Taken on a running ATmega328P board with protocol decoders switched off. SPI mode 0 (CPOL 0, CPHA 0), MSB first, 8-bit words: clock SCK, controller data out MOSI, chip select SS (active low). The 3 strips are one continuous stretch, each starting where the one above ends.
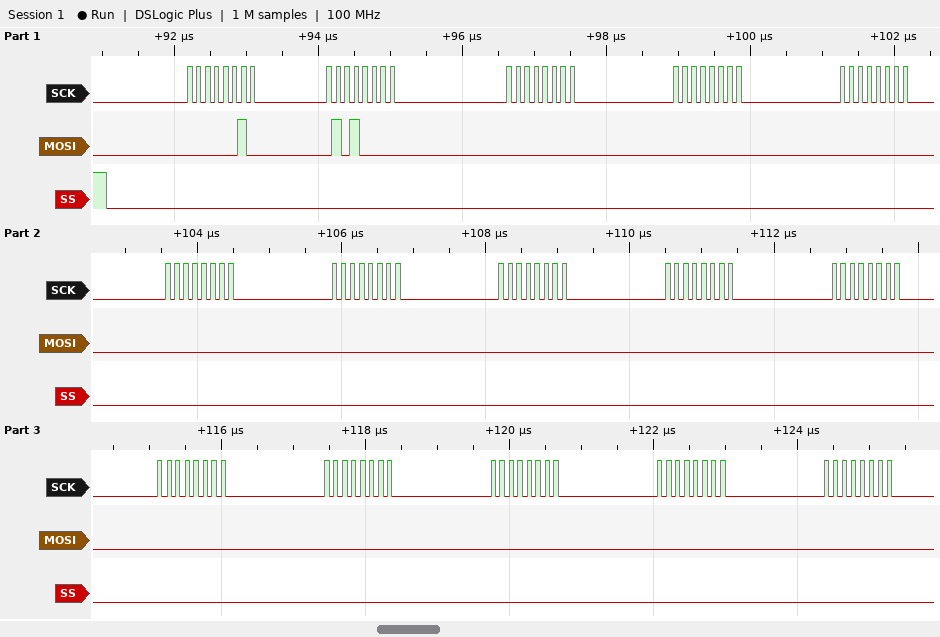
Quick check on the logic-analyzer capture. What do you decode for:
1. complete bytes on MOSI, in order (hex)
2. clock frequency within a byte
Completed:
02 50 00 00 00 00 00 00 00 00 00 00 00 00 00
8 MHz
